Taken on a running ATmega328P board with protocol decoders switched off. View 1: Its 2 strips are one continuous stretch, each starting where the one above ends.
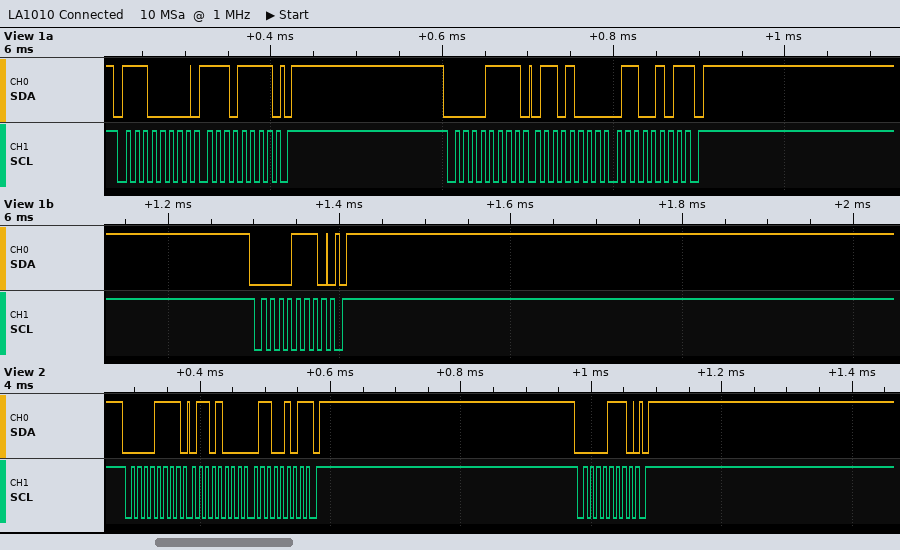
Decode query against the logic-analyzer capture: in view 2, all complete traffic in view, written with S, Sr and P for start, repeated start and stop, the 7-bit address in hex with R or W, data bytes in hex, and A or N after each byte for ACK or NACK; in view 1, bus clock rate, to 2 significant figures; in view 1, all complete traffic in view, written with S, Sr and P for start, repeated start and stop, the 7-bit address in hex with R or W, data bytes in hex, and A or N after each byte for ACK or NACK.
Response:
S 07R A 68 A 65 N P S 07W A P
100 kHz
S 70W A EF A P S 07R A 68 A 65 N P S 07W A P
